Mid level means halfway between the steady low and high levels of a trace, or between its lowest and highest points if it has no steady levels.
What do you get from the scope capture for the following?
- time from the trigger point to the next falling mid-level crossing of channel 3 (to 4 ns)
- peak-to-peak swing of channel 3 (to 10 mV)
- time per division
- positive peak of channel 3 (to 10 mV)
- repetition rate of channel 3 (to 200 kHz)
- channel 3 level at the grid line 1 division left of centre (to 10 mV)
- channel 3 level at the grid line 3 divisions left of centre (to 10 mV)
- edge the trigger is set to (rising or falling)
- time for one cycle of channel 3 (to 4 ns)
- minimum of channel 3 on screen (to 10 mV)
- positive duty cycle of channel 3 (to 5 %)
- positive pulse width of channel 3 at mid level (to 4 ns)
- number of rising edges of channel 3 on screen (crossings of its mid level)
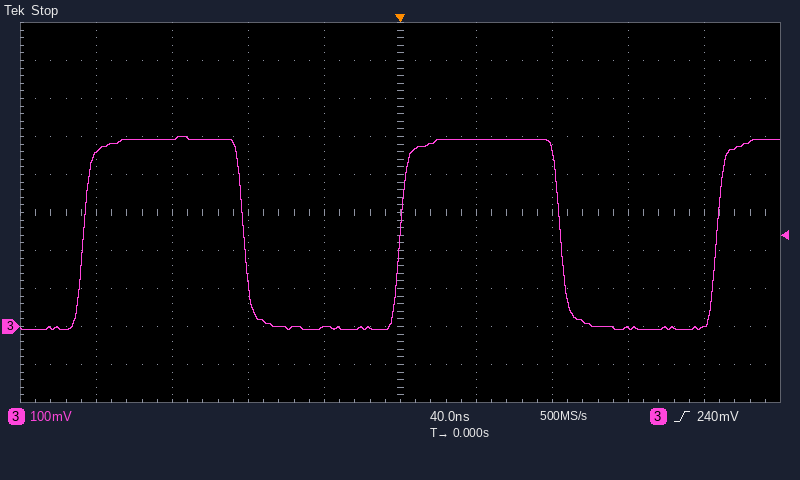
84 ns
510 mV
40 ns
500 mV
6.0 MHz
0 mV
490 mV
rising
168 ns
-10 mV
50 %
84 ns
3
